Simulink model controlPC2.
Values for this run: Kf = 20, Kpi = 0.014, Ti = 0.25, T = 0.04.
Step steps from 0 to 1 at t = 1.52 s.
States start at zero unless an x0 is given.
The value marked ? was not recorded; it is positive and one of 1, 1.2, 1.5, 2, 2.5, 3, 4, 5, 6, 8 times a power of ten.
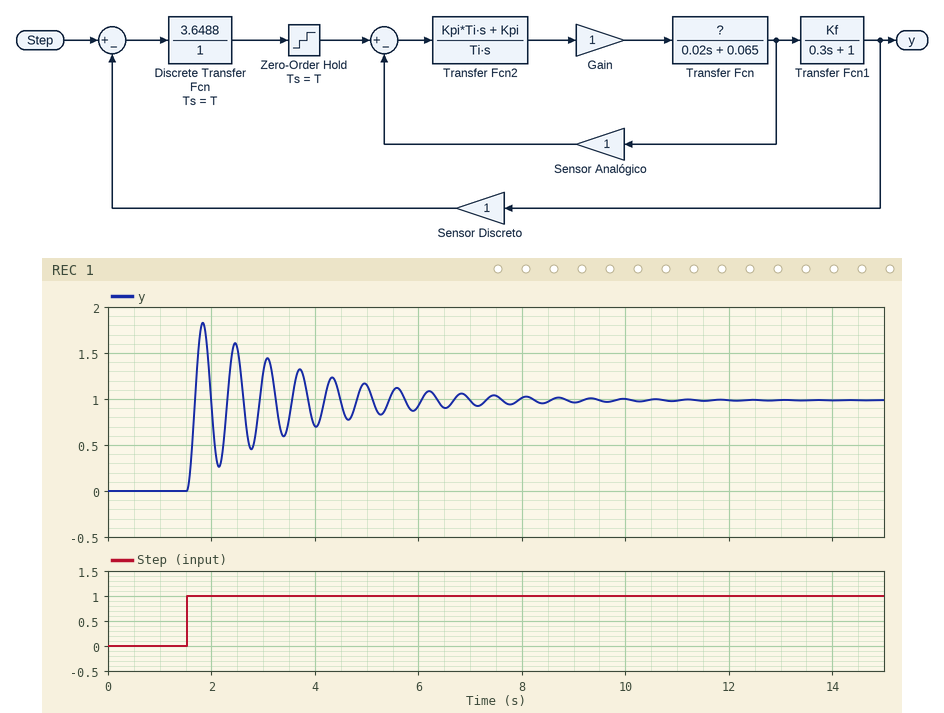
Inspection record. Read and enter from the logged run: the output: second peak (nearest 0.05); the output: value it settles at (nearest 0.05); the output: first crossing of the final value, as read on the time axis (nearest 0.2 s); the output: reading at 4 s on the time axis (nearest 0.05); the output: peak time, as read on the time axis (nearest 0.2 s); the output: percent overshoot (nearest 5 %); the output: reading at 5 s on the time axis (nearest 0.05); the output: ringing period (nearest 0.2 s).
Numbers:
1.60
1.00
1.6 s
0.70
1.8 s
85 %
1.15
0.6 s
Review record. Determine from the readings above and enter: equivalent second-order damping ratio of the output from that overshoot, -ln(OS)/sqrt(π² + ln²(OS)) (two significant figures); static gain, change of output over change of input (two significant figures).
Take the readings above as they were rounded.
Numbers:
0.052
1.0
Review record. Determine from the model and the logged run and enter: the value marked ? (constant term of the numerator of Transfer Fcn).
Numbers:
0.6
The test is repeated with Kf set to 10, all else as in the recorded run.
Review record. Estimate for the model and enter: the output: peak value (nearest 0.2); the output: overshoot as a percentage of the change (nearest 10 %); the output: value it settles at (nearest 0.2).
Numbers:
1.6
60 %
1.0
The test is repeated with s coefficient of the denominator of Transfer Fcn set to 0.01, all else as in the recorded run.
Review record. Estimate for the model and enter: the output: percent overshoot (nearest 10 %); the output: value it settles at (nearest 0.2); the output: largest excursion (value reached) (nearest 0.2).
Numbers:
80 %
1.0
1.8
